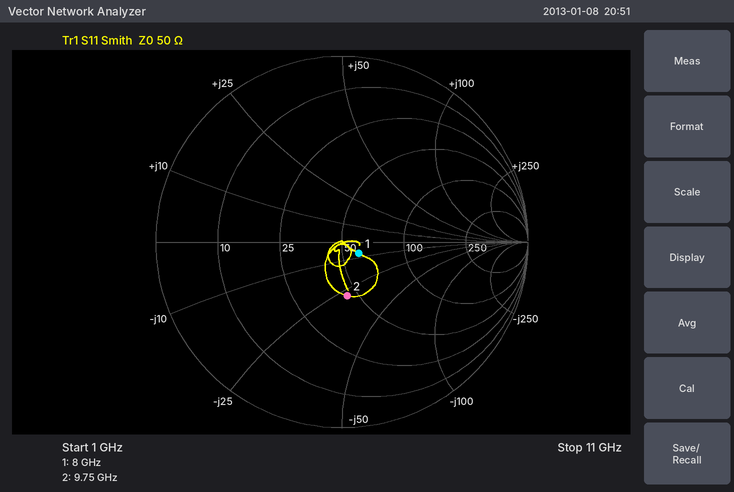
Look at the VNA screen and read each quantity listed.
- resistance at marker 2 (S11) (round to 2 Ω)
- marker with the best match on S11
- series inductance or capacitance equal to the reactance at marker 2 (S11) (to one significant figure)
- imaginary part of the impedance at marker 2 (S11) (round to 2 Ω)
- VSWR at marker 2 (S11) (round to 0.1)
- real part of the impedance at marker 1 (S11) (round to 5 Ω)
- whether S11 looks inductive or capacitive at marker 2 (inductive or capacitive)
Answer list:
44 Ω
marker 1
600 fF
-28 Ω
1.8
60 Ω
capacitive
